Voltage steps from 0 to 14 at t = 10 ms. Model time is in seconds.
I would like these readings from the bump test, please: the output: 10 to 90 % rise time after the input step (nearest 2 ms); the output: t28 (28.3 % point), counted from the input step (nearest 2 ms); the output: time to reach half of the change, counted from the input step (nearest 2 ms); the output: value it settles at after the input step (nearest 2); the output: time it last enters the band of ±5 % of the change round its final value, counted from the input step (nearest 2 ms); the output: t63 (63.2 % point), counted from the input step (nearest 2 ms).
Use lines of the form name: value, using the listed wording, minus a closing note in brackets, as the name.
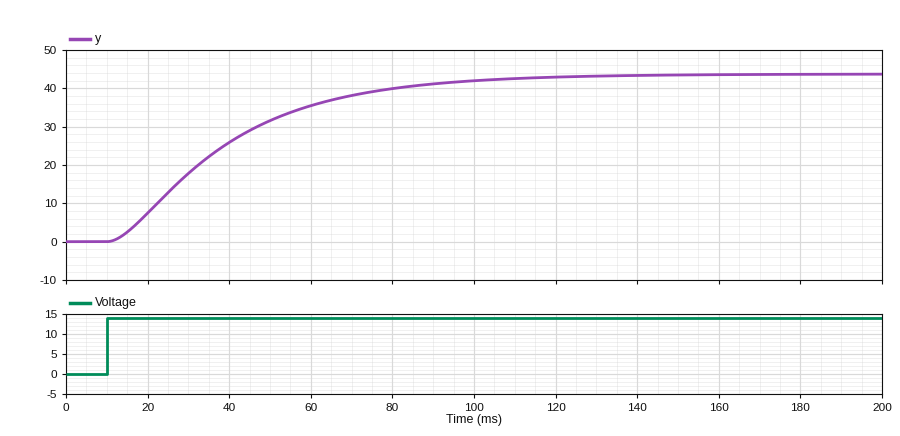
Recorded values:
the output: 10 to 90 % rise time after the input step: 60 ms
the output: t28 (28.3 % point), counted from the input step: 14 ms
the output: time to reach half of the change, counted from the input step: 24 ms
the output: value it settles at after the input step: 44
the output: time it last enters the band of ±5 % of the change round its final value, counted from the input step: 84 ms
the output: t63 (63.2 % point), counted from the input step: 32 ms
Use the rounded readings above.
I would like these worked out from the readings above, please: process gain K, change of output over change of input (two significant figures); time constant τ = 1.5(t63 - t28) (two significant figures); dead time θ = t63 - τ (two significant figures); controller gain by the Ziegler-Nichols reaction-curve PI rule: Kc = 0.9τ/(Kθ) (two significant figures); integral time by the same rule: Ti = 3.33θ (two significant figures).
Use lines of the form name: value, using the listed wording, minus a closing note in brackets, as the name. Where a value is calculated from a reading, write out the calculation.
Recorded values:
process gain K, change of output over change of input: (44 - 0) / 14 = 3.1
time constant τ = 1.5(t63 - t28): 1.5 × (32 - 14) = 27 ms
dead time θ = t63 - τ: 32 - 27 = 5.0 ms
controller gain by the Ziegler-Nichols reaction-curve PI rule: Kc = 0.9τ/(Kθ): 0.9 × 27 / (3.1 × 5) = 1.6
integral time by the same rule: Ti = 3.33θ: 3.33 × 5 = 17 ms
